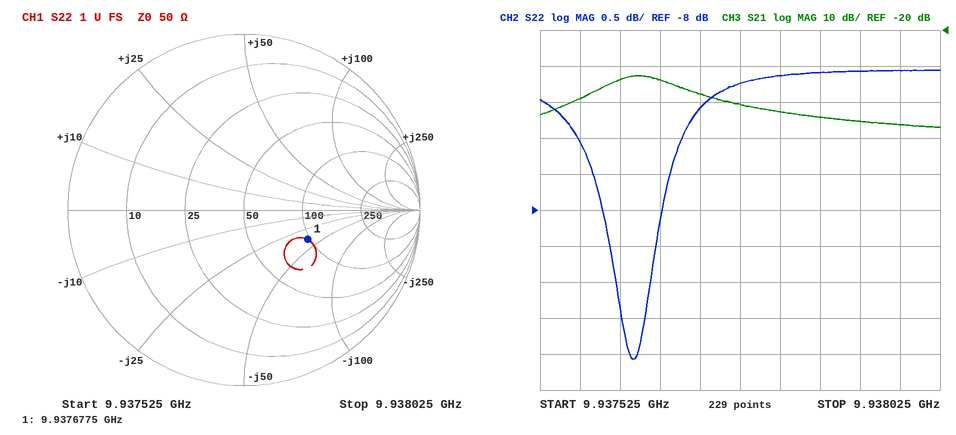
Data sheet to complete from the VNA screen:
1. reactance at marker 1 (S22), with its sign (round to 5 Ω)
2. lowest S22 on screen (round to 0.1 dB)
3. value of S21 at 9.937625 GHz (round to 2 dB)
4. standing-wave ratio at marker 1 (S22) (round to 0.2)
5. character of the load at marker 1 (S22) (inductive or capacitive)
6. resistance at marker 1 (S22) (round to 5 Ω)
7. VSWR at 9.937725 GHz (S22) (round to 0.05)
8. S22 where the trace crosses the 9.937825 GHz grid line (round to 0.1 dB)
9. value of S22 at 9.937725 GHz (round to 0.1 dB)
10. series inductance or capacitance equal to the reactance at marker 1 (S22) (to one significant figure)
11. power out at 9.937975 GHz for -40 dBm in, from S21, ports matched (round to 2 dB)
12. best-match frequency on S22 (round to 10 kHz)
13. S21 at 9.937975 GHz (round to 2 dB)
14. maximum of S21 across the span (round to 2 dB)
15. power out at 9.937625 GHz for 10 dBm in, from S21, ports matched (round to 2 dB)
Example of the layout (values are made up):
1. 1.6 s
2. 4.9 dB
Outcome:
1. -40 Ω
2. -10.1 dB
3. -34 dB
4. 2.4
5. capacitive
6. 95 Ω
7. 2.75
8. -6.1 dB
9. -6.6 dB
10. 400 fF
11. -86 dBm
12. 9.93764 GHz
13. -46 dB
14. -32 dB
15. -24 dBm
